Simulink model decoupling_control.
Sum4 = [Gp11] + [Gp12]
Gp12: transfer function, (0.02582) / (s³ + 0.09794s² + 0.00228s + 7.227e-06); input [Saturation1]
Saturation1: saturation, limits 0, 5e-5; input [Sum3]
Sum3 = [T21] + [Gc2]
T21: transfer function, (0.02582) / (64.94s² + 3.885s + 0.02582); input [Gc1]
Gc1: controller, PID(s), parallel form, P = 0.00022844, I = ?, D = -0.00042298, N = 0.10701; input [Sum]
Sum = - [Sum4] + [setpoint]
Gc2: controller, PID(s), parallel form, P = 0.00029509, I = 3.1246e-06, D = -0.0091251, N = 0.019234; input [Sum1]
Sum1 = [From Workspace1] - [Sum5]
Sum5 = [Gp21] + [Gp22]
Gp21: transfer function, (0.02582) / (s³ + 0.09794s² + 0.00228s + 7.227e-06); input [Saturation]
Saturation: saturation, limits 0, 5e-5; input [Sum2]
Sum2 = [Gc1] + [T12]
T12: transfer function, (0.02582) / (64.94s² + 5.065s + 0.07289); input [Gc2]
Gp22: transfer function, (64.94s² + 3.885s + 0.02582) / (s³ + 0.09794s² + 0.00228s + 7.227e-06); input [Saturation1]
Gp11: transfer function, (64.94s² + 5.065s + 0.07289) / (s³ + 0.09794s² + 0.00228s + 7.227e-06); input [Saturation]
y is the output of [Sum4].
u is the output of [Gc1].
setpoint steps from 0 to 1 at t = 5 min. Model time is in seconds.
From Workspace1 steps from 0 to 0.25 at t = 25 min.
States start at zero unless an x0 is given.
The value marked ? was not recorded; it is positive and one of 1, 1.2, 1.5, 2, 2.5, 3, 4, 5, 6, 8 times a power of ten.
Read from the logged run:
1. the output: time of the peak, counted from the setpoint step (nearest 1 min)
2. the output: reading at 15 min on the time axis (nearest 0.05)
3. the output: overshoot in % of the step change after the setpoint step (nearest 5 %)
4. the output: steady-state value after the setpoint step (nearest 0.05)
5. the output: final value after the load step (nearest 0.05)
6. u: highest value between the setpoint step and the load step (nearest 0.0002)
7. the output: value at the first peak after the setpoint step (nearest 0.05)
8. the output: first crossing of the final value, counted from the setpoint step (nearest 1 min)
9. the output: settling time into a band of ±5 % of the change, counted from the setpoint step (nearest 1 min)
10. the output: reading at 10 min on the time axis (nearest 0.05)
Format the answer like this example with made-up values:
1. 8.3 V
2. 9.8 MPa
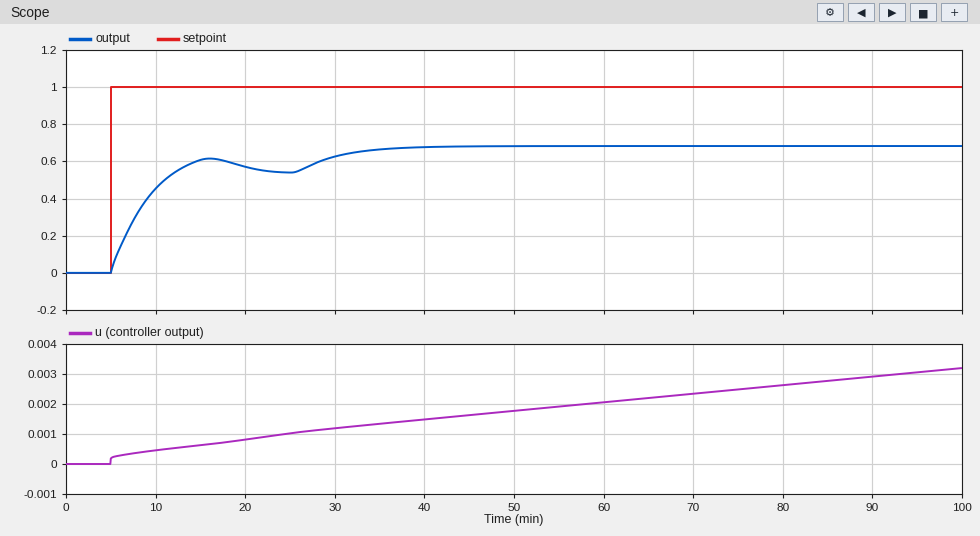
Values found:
1. 11 min
2. 0.60
3. 15 %
4. 0.55
5. 0.70
6. 0.0010
7. 0.60
8. 7 min
9. 15 min
10. 0.45
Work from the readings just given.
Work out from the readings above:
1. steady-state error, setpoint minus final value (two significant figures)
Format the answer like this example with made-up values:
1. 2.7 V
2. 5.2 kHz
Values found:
1. 0.45
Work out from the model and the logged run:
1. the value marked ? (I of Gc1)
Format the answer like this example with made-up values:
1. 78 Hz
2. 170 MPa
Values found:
1. 1.5e-06
